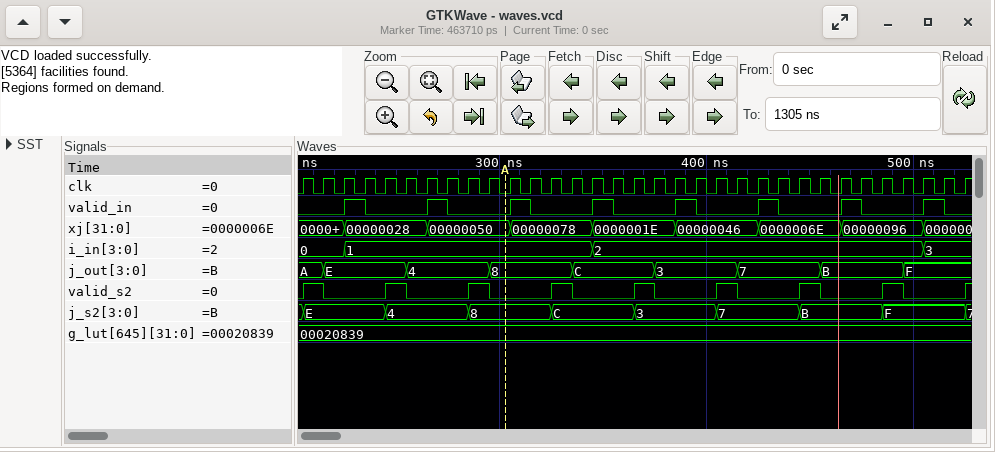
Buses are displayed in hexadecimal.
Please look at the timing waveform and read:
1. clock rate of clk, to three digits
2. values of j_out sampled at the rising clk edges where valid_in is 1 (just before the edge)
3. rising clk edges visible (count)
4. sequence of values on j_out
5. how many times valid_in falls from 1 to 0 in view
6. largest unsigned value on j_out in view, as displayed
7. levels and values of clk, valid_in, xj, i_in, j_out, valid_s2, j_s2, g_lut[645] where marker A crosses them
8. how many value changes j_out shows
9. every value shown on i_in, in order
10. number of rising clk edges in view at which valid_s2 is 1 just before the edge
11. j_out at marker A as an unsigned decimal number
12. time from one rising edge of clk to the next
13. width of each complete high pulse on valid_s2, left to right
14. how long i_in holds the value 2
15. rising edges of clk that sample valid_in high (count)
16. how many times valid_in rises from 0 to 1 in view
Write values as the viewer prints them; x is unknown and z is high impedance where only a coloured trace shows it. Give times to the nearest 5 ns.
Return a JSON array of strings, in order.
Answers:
["100 MHz", "E, 4, 8, C, 3, 7, B, F", "33", "A, E, 4, 8, C, 3, 7, B, F", "8", "F", "clk=0, valid_in=0, xj=00000050, i_in=1, j_out=8, valid_s2=0, j_s2=8, g_lut[645]=00020839", "8", "0, 1, 2, 3", "8", "8", "10 ns", "10 ns, 10 ns, 10 ns, 10 ns, 10 ns, 10 ns, 10 ns, 10 ns", "160 ns", "8", "8"]
